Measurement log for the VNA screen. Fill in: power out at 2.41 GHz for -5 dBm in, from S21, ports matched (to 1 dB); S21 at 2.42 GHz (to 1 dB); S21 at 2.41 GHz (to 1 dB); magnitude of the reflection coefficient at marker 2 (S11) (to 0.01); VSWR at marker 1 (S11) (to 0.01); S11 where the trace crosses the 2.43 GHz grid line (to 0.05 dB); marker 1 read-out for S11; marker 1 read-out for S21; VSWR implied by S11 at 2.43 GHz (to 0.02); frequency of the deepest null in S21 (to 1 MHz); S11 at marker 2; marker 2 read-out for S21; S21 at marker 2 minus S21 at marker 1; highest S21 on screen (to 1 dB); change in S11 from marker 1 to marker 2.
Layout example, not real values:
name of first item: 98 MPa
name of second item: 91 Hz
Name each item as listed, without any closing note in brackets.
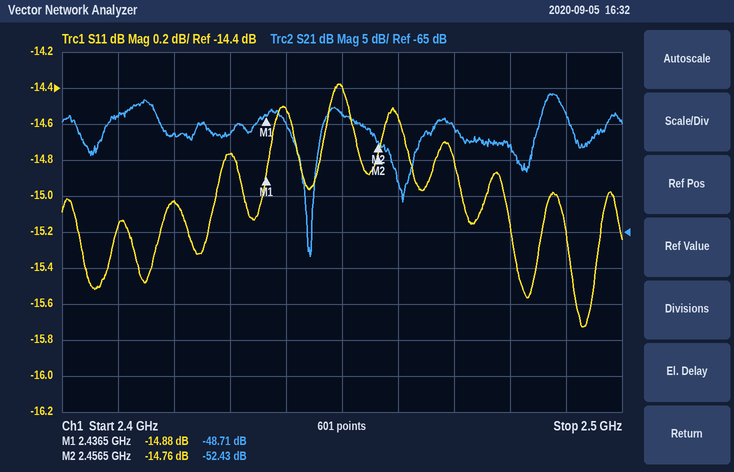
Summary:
power out at 2.41 GHz for -5 dBm in, from S21, ports matched: -54 dBm
S21 at 2.42 GHz: -51 dB
S21 at 2.41 GHz: -49 dB
magnitude of the reflection coefficient at marker 2 (S11): 0.18
VSWR at marker 1 (S11): 1.44
S11 where the trace crosses the 2.43 GHz grid line: -14.75 dB
marker 1 read-out for S11: -14.88 dB
marker 1 read-out for S21: -48.71 dB
VSWR implied by S11 at 2.43 GHz: 1.44
frequency of the deepest null in S21: 2.444 GHz
S11 at marker 2: -14.76 dB
marker 2 read-out for S21: -52.43 dB
S21 at marker 2 minus S21 at marker 1: -3.72 dB
highest S21 on screen: -46 dB
change in S11 from marker 1 to marker 2: 0.12 dB
